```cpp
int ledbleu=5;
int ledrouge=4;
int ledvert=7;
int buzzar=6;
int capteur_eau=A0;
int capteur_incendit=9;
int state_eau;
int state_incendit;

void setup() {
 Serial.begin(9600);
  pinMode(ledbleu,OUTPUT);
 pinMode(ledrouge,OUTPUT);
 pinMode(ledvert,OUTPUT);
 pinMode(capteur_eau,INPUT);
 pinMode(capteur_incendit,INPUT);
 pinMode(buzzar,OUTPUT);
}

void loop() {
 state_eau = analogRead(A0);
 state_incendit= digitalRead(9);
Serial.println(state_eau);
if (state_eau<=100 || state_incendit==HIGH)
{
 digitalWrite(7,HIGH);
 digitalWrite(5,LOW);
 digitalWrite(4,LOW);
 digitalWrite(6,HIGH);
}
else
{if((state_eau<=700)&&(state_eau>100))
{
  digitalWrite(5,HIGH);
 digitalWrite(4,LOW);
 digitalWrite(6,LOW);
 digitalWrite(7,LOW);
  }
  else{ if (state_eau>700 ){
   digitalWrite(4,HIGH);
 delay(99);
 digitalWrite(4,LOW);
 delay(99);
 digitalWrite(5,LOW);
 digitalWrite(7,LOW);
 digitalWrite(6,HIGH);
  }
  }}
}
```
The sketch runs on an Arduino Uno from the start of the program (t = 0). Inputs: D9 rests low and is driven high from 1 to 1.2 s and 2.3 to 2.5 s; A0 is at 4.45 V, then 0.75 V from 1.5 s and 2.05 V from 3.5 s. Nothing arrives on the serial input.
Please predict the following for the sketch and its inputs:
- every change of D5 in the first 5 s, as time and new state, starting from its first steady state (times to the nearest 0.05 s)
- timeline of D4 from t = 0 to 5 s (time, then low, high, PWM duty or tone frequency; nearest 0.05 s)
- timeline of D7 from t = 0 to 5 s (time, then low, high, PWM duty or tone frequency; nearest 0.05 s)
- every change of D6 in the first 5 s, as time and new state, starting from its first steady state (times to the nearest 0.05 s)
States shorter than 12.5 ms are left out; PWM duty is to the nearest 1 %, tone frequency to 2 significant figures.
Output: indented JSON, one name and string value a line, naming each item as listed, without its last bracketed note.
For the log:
{
  "every change of D5 in the first 5 s, as time and new state, starting from its first steady state": "0 s low; 1.6 s high; 2.3 s low; 2.5 s high",
  "timeline of D4 from t = 0 to 5 s": "0 s high; 0.1 s low; 0.2 s high; 0.3 s low; 0.4 s high; 0.5 s low; 0.6 s high; 0.7 s low; 0.8 s high; 0.9 s low; 1 s high; 1.1 s low; 1.2 s high; 1.3 s low; 1.4 s high; 1.5 s low",
  "timeline of D7 from t = 0 to 5 s": "0 s low; 1.2 s high; 1.4 s low; 2.3 s high; 2.5 s low",
  "every change of D6 in the first 5 s, as time and new state, starting from its first steady state": "0 s low; 0.2 s high; 1.6 s low; 2.3 s high; 2.5 s low"
}
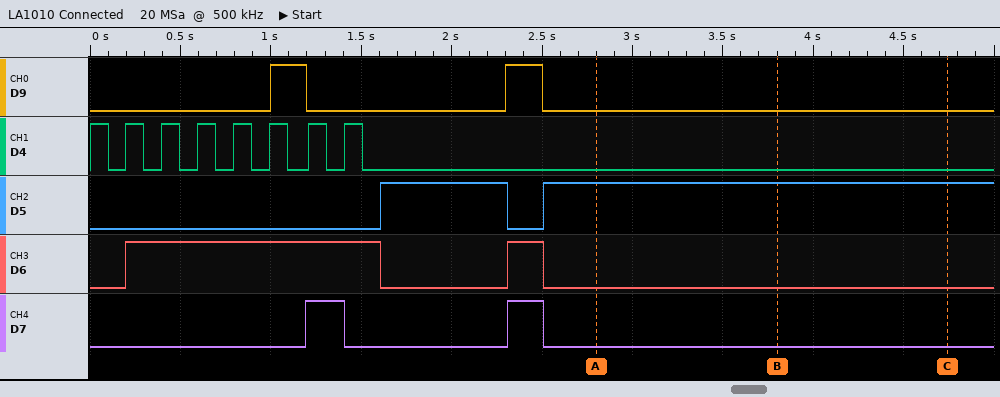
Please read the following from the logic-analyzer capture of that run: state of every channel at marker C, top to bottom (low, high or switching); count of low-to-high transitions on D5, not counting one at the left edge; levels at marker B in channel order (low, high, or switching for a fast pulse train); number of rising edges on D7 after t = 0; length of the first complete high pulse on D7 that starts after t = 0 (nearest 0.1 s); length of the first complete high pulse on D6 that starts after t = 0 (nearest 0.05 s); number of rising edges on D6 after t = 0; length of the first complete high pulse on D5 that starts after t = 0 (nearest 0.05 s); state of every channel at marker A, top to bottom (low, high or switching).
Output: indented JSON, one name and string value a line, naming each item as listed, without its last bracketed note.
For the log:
{
  "state of every channel at marker C, top to bottom": "D9 low, D4 low, D5 high, D6 low, D7 low",
  "count of low-to-high transitions on D5, not counting one at the left edge": "2",
  "levels at marker B in channel order": "D9 low, D4 low, D5 high, D6 low, D7 low",
  "number of rising edges on D7 after t = 0": "2",
  "length of the first complete high pulse on D7 that starts after t = 0": "0.2 s",
  "length of the first complete high pulse on D6 that starts after t = 0": "1.40 s",
  "number of rising edges on D6 after t = 0": "2",
  "length of the first complete high pulse on D5 that starts after t = 0": "0.70 s",
  "state of every channel at marker A, top to bottom": "D9 low, D4 low, D5 high, D6 low, D7 low"
}
